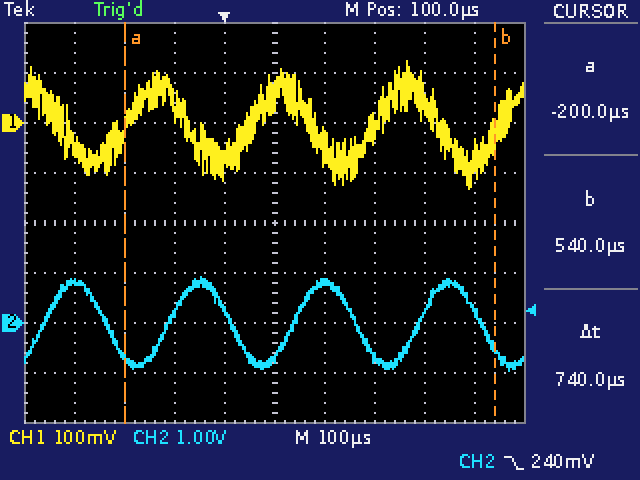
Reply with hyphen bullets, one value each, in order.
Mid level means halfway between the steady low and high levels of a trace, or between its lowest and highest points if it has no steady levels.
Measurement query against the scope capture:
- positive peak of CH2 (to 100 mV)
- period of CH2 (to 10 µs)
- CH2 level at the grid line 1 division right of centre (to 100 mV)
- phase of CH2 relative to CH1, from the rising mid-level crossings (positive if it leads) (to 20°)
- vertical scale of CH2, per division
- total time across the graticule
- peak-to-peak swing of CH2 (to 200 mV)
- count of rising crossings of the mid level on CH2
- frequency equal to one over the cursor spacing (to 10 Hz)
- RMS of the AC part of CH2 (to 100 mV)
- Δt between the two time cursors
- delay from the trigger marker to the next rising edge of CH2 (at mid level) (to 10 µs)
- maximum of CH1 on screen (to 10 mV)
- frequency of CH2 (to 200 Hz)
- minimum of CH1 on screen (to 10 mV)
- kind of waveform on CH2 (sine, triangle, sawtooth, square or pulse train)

- 900 mV
- 250 µs
- 800 mV
- -120°
- 1 V
- 1 ms
- 1.8 V
- 4
- 1.35 kHz
- 600 mV
- 740 µs
- 140 µs
- 120 mV
- 4.0 kHz
- -130 mV
- sine
